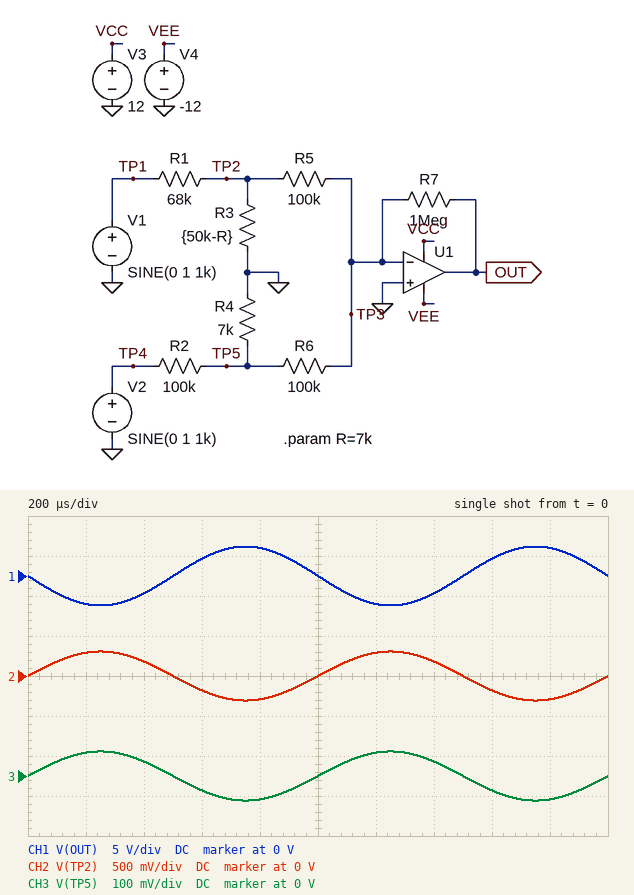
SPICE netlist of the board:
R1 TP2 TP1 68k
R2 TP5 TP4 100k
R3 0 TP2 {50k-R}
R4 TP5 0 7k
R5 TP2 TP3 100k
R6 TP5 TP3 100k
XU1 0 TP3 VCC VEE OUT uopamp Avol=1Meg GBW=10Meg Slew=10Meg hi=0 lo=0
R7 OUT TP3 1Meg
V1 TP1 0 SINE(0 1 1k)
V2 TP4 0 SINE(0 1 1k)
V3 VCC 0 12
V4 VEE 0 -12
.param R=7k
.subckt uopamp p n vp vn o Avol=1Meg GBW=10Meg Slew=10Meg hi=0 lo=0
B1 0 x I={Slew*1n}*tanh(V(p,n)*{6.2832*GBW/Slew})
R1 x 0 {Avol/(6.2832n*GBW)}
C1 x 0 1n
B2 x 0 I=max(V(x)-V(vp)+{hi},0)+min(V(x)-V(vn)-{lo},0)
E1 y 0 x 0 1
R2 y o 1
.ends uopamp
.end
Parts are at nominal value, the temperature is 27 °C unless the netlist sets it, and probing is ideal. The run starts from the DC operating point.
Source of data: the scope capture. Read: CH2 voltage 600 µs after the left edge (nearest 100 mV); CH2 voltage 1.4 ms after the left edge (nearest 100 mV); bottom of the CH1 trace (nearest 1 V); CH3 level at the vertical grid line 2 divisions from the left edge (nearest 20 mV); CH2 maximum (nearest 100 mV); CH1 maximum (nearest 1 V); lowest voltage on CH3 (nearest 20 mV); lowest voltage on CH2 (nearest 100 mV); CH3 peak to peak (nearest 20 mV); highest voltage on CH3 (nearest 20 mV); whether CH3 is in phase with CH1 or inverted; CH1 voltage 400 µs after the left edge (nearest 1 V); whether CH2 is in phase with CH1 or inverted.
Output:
-200 mV
200 mV
-4 V
40 mV
300 mV
4 V
-60 mV
-300 mV
120 mV
60 mV
inverted
-2 V
inverted
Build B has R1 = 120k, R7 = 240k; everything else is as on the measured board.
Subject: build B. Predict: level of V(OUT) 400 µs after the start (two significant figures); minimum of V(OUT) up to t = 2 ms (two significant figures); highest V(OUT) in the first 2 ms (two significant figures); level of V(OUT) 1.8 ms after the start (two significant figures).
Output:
-370 mV
-630 mV
630 mV
600 mV
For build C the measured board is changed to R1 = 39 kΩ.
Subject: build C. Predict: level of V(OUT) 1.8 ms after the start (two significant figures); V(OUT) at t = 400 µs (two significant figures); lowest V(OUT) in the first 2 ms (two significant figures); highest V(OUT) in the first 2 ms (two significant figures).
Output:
4.7 V
-2.9 V
-5.0 V
5.0 V
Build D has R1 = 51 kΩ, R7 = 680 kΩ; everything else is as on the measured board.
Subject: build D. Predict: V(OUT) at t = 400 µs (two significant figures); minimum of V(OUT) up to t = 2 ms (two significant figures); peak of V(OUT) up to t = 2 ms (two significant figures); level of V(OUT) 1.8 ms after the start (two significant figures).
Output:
-1.7 V
-2.9 V
2.9 V
2.8 V
